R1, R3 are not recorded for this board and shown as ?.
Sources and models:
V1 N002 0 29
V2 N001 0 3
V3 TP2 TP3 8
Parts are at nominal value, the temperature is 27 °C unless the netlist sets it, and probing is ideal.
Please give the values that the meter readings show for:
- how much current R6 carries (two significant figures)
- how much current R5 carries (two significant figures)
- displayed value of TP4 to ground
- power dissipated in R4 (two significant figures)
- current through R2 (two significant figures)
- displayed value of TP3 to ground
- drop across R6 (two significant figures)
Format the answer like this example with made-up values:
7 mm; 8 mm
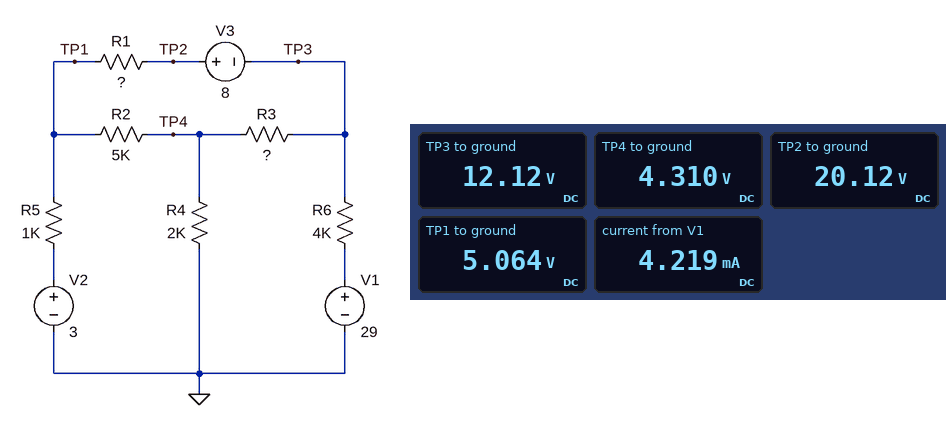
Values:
4.2 mA; 2.1 mA; 4.310 V; 9.3 mW; 150 µA; 12.12 V; 17 V
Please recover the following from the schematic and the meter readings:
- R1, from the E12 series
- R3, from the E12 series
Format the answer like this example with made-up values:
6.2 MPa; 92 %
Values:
6.8 kΩ; 3.9 kΩ
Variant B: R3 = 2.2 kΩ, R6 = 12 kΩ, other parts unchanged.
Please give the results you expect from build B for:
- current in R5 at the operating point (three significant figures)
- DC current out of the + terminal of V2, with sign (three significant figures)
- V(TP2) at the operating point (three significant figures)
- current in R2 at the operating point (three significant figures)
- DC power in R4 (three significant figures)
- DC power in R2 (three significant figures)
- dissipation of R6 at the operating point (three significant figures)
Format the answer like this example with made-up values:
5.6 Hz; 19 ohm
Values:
904 µA; -904 µA; 12.2 V; 315 µA; 2.71 mW; 497 µW; 51.3 mW
